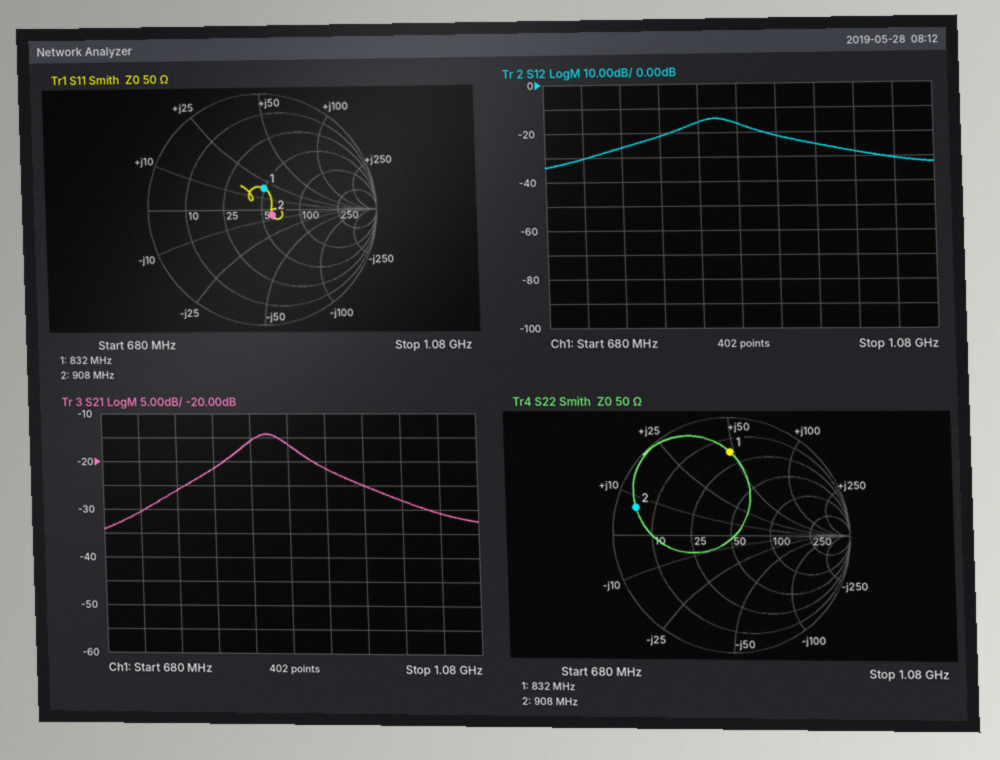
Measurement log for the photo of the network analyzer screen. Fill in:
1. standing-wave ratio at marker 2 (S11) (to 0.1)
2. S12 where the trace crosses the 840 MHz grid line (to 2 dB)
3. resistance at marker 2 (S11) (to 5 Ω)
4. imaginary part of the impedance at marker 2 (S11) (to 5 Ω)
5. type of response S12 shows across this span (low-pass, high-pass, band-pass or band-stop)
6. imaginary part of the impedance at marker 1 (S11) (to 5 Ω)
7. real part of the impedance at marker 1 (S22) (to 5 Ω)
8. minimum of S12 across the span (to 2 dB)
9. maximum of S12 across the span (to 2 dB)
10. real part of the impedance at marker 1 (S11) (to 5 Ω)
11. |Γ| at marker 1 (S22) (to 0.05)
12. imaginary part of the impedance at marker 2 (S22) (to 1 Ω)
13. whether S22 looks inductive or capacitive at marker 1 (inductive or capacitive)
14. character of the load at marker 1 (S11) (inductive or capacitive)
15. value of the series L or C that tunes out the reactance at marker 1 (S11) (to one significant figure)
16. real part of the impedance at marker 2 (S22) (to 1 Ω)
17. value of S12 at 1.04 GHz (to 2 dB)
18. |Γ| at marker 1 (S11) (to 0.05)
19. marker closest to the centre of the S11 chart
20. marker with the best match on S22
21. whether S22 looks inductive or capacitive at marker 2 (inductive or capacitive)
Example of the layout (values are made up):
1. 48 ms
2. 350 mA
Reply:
1. 1.2
2. -16 dB
3. 60 Ω
4. -5 Ω
5. band-pass
6. +20 Ω
7. 15 Ω
8. -34 dB
9. -14 dB
10. 50 Ω
11. 0.70
12. +7 Ω
13. inductive
14. inductive
15. 10 pF
16. 5 Ω
17. -30 dB
18. 0.20
19. marker 2
20. marker 1
21. inductive
